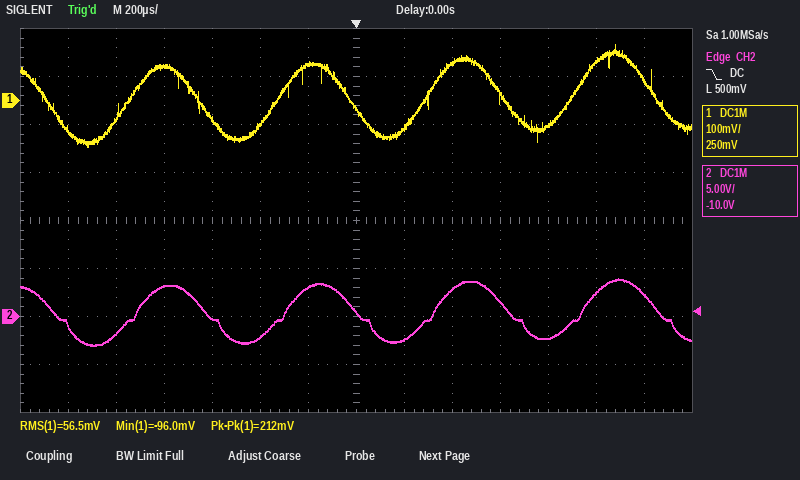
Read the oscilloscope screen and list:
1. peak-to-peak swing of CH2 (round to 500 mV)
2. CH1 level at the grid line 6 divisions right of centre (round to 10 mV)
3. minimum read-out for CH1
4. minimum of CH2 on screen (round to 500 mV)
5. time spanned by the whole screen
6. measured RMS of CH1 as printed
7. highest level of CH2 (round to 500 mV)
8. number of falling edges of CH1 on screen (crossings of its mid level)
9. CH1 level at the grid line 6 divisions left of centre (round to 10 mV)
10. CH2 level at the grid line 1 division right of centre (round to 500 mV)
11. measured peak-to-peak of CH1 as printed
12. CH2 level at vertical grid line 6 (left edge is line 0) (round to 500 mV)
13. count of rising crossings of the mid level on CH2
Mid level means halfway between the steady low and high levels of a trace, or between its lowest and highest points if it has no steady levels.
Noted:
7.0 V
40 mV
-96.0 mV
-3.0 V
2.8 ms
56.5 mV
4.0 V
5
-60 mV
-2.5 V
212 mV
3.0 V
4
